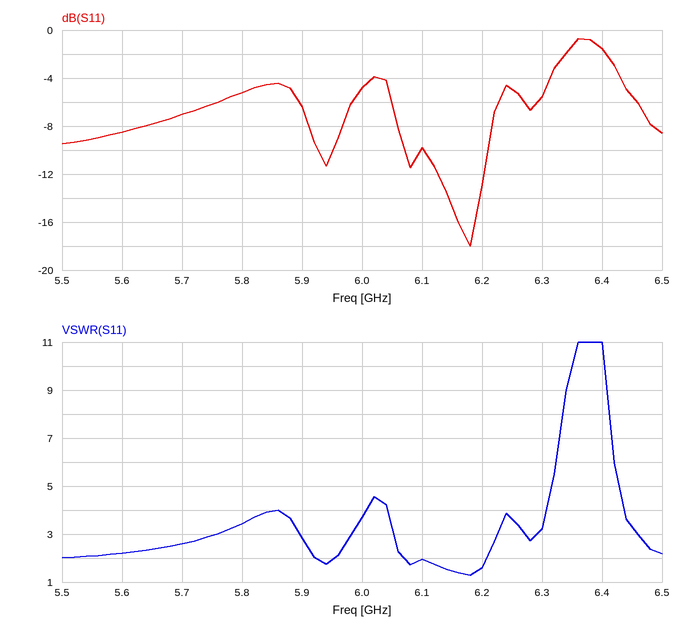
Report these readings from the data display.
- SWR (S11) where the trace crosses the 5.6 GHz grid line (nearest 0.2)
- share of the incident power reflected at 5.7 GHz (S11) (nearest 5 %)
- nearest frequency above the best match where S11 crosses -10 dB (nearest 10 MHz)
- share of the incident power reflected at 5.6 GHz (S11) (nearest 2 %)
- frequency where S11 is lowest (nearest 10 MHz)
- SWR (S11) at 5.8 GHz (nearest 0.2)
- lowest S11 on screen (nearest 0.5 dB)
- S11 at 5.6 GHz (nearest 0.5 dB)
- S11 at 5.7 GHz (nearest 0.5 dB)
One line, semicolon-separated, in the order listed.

2.2; 20 %; 6.21 GHz; 14 %; 6.18 GHz; 3.4; -18.0 dB; -8.5 dB; -7.0 dB
